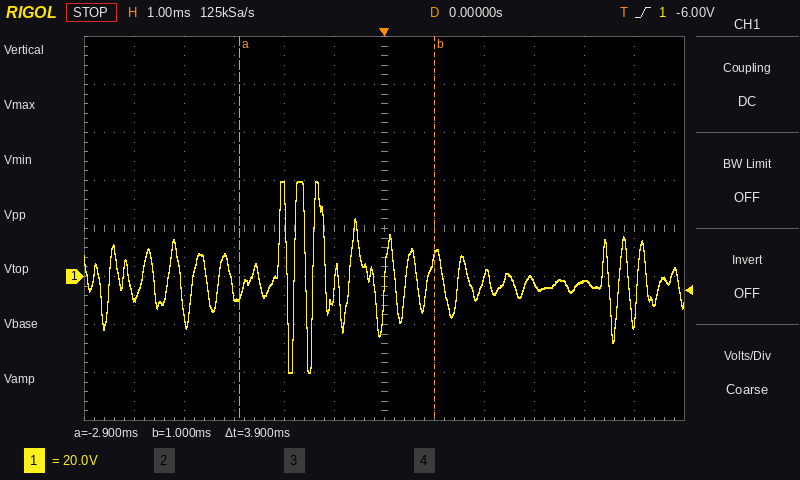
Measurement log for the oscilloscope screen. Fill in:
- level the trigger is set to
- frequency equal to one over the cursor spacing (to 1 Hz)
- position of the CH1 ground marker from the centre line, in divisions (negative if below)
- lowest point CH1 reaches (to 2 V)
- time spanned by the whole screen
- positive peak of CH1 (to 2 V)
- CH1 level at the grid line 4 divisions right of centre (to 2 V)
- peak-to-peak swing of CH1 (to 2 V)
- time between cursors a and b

-6.00 V
256 Hz
-1.0 div
-40 V
12 ms
40 V
-2 V
80 V
3.9 ms
